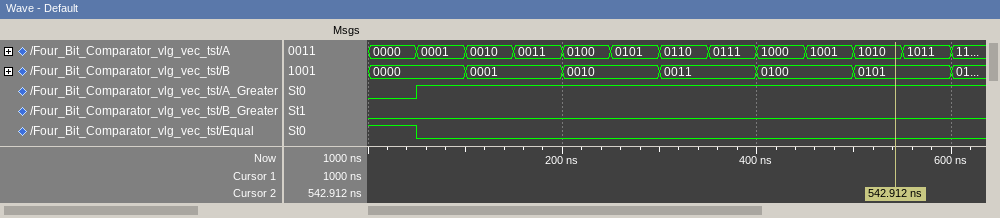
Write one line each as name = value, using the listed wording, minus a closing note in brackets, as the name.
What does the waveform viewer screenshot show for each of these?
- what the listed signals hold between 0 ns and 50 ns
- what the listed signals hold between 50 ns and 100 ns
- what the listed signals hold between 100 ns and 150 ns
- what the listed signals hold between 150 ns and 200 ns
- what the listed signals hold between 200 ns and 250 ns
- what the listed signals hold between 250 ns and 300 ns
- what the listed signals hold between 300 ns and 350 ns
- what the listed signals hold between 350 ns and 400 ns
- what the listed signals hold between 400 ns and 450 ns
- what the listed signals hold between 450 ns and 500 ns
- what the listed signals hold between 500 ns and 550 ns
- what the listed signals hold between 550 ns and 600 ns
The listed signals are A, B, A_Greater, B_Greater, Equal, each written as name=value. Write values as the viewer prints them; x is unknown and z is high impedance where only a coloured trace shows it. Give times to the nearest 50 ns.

what the listed signals hold between 0 ns and 50 ns = A=0000, B=0000, A_Greater=0, B_Greater=0, Equal=1
what the listed signals hold between 50 ns and 100 ns = A=0001, B=0000, A_Greater=1, B_Greater=0, Equal=0
what the listed signals hold between 100 ns and 150 ns = A=0010, B=0001, A_Greater=1, B_Greater=0, Equal=0
what the listed signals hold between 150 ns and 200 ns = A=0011, B=0001, A_Greater=1, B_Greater=0, Equal=0
what the listed signals hold between 200 ns and 250 ns = A=0100, B=0010, A_Greater=1, B_Greater=0, Equal=0
what the listed signals hold between 250 ns and 300 ns = A=0101, B=0010, A_Greater=1, B_Greater=0, Equal=0
what the listed signals hold between 300 ns and 350 ns = A=0110, B=0011, A_Greater=1, B_Greater=0, Equal=0
what the listed signals hold between 350 ns and 400 ns = A=0111, B=0011, A_Greater=1, B_Greater=0, Equal=0
what the listed signals hold between 400 ns and 450 ns = A=1000, B=0100, A_Greater=1, B_Greater=0, Equal=0
what the listed signals hold between 450 ns and 500 ns = A=1001, B=0100, A_Greater=1, B_Greater=0, Equal=0
what the listed signals hold between 500 ns and 550 ns = A=1010, B=0101, A_Greater=1, B_Greater=0, Equal=0
what the listed signals hold between 550 ns and 600 ns = A=1011, B=0101, A_Greater=1, B_Greater=0, Equal=0
